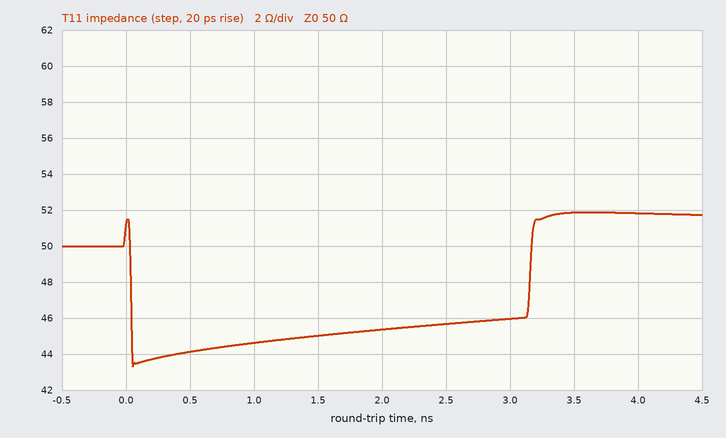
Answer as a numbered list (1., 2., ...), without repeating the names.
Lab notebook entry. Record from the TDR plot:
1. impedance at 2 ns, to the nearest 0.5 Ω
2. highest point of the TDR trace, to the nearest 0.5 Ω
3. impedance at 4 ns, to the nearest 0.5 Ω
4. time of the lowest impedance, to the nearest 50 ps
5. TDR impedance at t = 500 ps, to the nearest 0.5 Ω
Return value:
1. 45.5 Ω
2. 52.0 Ω
3. 52.0 Ω
4. 50 ps
5. 44.0 Ω
